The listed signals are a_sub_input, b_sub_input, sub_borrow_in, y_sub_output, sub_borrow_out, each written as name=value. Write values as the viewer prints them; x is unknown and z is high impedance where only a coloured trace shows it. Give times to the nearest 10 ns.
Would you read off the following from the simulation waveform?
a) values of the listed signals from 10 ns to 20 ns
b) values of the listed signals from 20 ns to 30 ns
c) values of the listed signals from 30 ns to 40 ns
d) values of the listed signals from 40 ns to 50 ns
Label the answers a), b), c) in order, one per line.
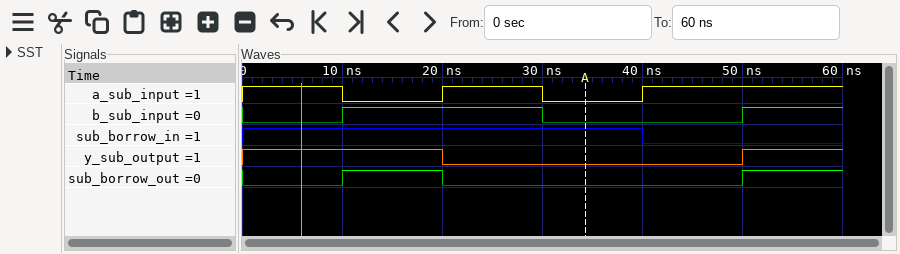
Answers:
a) a_sub_input=0, b_sub_input=1, sub_borrow_in=1, y_sub_output=1, sub_borrow_out=1
b) a_sub_input=1, b_sub_input=1, sub_borrow_in=1, y_sub_output=0, sub_borrow_out=0
c) a_sub_input=0, b_sub_input=0, sub_borrow_in=1, y_sub_output=0, sub_borrow_out=0
d) a_sub_input=1, b_sub_input=0, sub_borrow_in=0, y_sub_output=0, sub_borrow_out=0
